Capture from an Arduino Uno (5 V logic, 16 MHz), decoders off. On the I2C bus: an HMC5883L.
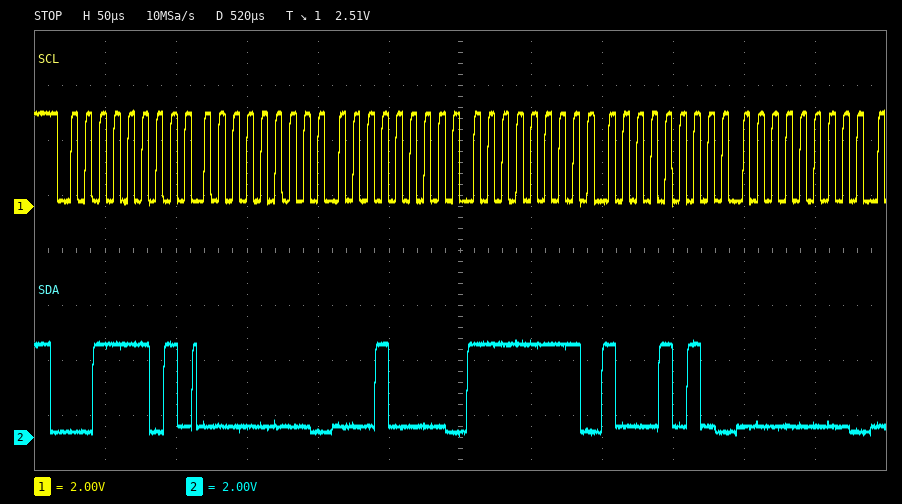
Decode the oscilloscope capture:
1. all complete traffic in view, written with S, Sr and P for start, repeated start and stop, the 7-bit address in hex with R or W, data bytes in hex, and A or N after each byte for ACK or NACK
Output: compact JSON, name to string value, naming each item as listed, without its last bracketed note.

{"all complete traffic in view, written with S, Sr and P for start, repeated start and stop, the 7-bit address in hex with R or W, data bytes in hex, and A or N after each byte for ACK or NACK": "S 1ER A 00 A 10 A FF A 8A A 00 A"}
